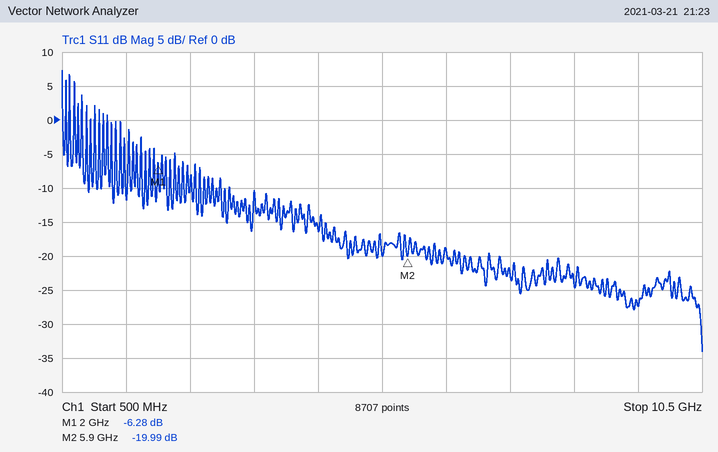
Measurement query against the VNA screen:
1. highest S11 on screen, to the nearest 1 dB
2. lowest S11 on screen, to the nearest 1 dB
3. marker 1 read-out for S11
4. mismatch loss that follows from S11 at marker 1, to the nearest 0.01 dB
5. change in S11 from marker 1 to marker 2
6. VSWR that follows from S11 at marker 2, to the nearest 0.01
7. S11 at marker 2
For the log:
7 dB
-34 dB
-6.28 dB
1.17 dB
-13.71 dB
1.22
-19.99 dB
